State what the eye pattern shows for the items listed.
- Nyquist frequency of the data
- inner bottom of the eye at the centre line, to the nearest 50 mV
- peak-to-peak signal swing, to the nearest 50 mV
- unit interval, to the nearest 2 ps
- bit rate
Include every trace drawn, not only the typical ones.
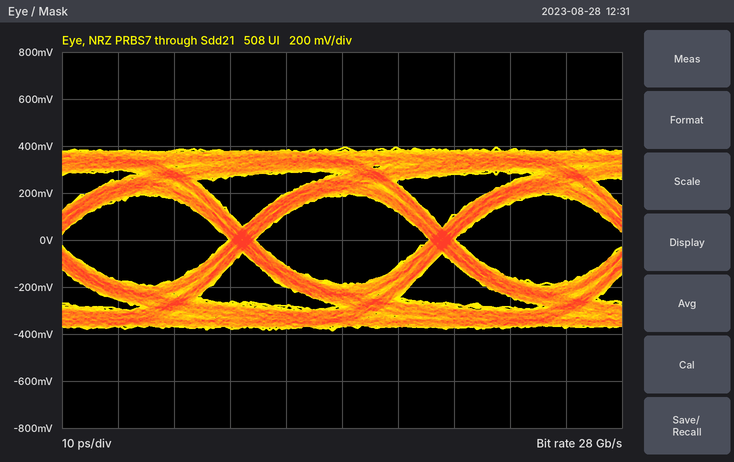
14 GHz
-200 mV
800 mV
36 ps
28 Gb/s
